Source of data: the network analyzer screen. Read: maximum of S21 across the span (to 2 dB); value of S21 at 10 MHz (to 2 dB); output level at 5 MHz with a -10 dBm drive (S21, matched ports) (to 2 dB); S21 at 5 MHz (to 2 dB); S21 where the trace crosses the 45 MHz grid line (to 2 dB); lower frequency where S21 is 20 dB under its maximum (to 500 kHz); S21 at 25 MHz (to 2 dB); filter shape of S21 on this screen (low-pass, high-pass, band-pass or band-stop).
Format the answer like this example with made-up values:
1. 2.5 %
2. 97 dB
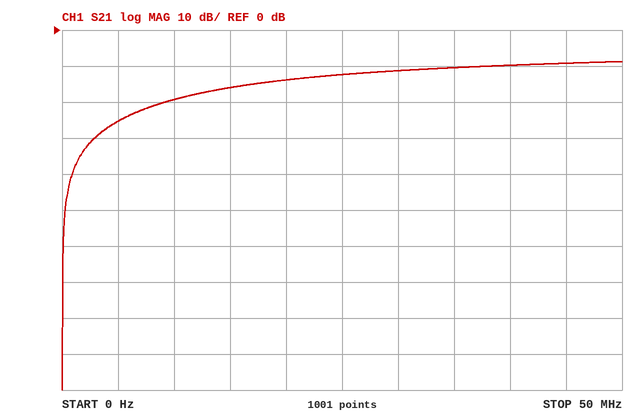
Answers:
1. -8 dB
2. -20 dB
3. -36 dBm
4. -26 dB
5. -10 dB
6. 3.5 MHz
7. -12 dB
8. high-pass
